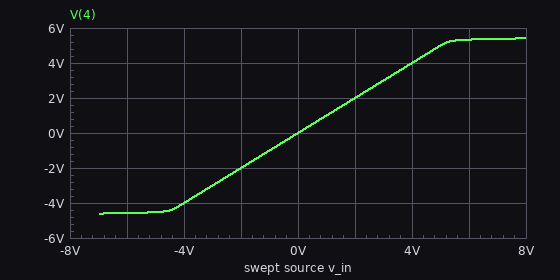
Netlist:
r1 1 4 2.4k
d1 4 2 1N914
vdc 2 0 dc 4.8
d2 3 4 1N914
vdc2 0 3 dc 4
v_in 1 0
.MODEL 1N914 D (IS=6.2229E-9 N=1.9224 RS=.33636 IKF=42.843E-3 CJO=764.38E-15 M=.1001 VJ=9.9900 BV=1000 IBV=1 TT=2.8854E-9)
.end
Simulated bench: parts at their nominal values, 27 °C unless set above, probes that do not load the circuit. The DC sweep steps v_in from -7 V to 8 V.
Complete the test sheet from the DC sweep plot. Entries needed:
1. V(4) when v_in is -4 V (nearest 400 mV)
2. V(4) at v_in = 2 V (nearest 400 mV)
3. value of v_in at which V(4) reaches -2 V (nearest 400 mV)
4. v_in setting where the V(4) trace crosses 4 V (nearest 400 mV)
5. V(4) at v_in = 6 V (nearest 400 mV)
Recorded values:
-4.0 V
2.0 V
-2.0 V
4.0 V
5.2 V
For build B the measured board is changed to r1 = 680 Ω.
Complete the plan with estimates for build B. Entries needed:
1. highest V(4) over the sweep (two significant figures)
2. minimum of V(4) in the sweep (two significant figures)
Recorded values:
5.5 V
-4.7 V
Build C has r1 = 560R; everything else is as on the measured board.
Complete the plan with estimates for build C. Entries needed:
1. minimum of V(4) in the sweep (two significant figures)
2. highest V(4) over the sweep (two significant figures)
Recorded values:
-4.7 V
5.5 V
